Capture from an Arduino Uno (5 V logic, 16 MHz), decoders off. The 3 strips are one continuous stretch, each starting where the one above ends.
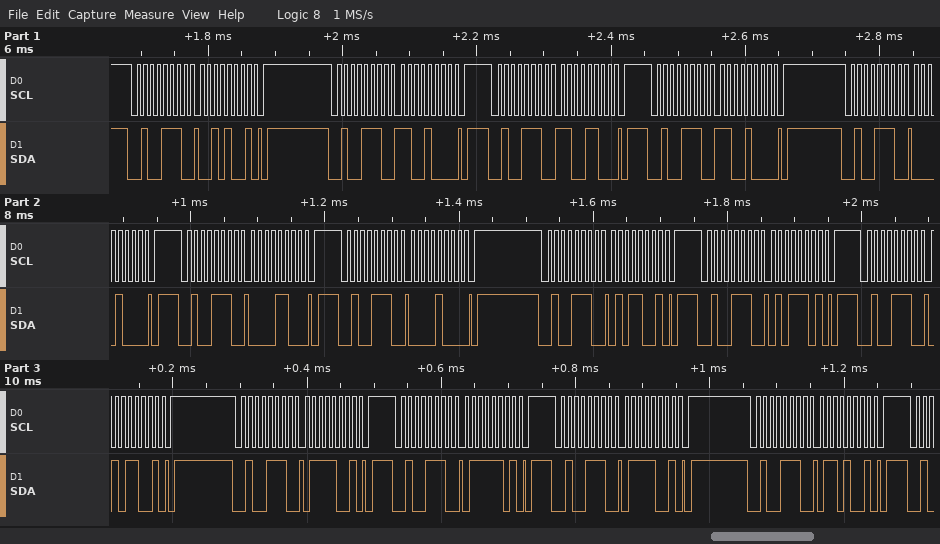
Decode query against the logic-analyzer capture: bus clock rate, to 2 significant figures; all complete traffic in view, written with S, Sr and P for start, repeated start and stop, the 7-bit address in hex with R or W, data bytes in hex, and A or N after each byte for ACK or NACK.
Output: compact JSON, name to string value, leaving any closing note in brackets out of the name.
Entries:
{"bus clock rate, to 2 significant figures": "100 kHz", "all complete traffic in view, written with S, Sr and P for start, repeated start and stop, the 7-bit address in hex with R or W, data bytes in hex, and A or N after each byte for ACK or NACK": "S 27W A 29 A P S 27W A C8 A P S 27W A CC A P S 27W A C8 A P S 27W A 08 A P S 27W A 0C A P S 27W A 08 A P S 27W A 59 A P S 27W A 5D A P S 27W A 59 A P S 27W A 79 A P S 27W A 7D A P S 27W A 79 A P S 27W A 69 A P"}
